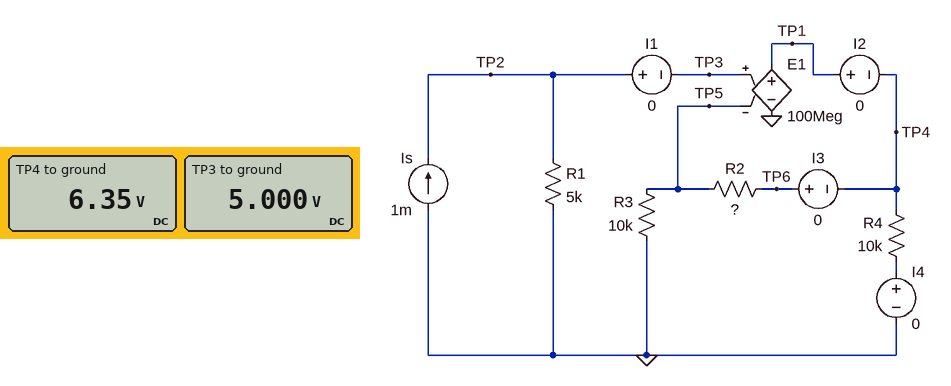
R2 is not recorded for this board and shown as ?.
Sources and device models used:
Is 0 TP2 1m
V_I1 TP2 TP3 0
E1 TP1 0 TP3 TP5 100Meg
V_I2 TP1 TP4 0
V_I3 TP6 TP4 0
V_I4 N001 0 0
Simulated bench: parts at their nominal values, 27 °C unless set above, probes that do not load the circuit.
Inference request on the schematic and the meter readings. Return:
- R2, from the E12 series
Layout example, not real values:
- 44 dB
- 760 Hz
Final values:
- 2.7 kΩ
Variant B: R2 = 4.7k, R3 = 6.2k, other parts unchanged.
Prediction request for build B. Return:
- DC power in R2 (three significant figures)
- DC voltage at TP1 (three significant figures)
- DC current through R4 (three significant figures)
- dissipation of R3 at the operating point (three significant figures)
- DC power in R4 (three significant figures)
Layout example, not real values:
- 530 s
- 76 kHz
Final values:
- 3.06 mW
- 8.79 V
- 879 µA
- 4.03 mW
- 7.73 mW
